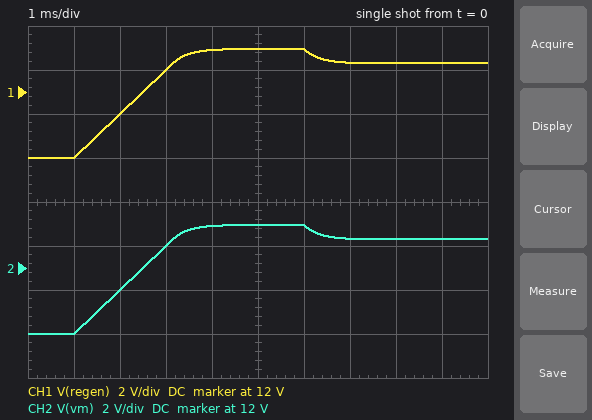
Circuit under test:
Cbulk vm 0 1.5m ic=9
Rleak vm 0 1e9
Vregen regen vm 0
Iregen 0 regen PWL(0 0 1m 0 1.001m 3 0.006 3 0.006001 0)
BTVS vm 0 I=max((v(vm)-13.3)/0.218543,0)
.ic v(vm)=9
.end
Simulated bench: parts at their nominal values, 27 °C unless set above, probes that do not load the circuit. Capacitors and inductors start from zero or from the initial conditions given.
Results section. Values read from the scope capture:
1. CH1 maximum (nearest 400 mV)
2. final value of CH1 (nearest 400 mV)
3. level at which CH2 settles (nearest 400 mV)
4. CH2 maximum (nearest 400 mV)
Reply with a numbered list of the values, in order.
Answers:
1. 14.0 V
2. 13.2 V
3. 13.2 V
4. 14.0 V
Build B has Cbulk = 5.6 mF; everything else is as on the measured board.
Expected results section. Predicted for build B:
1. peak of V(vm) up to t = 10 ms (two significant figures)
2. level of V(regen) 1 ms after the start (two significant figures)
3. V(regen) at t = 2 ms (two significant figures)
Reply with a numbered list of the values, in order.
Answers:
1. 12 V
2. 9.0 V
3. 9.5 V
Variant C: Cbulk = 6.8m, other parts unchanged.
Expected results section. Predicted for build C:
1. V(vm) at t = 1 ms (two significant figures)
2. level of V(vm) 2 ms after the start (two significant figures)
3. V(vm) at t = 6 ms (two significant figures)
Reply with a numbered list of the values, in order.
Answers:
1. 9.0 V
2. 9.4 V
3. 11 V
